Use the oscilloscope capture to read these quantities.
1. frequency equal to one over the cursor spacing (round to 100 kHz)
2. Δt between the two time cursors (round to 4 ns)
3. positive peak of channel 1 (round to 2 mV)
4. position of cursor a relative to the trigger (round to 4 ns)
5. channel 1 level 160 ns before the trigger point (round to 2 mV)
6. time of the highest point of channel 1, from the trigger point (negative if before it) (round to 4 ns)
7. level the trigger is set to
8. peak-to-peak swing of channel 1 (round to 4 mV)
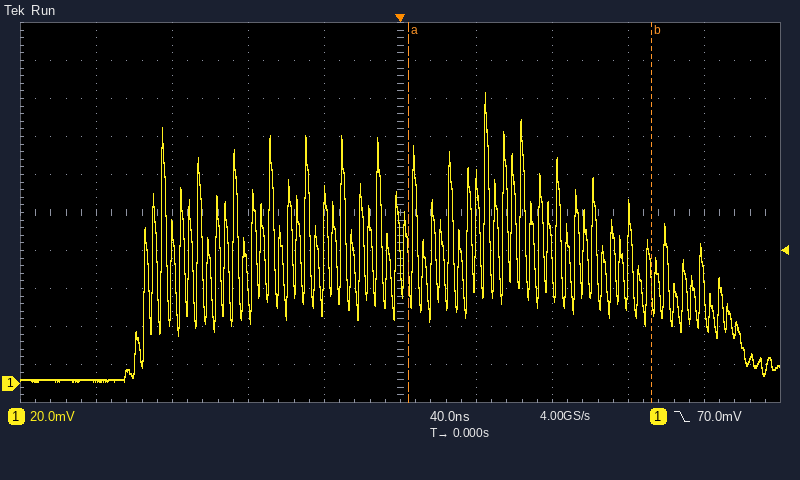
7.8 MHz
128 ns
154 mV
+4 ns
2 mV
+44 ns
70.0 mV
152 mV
